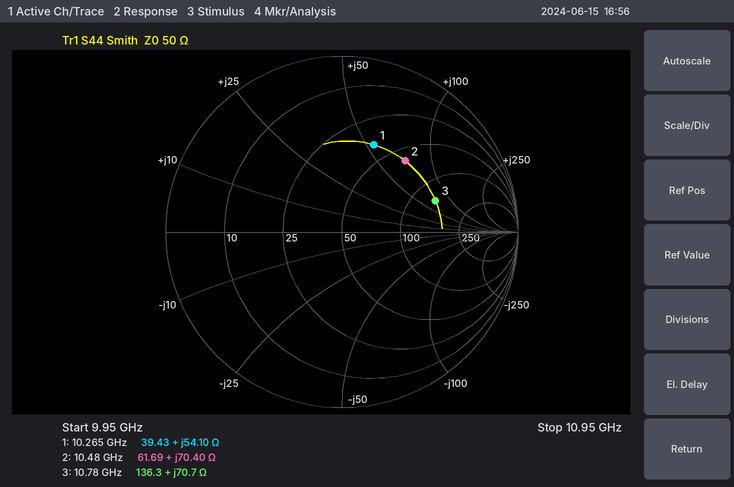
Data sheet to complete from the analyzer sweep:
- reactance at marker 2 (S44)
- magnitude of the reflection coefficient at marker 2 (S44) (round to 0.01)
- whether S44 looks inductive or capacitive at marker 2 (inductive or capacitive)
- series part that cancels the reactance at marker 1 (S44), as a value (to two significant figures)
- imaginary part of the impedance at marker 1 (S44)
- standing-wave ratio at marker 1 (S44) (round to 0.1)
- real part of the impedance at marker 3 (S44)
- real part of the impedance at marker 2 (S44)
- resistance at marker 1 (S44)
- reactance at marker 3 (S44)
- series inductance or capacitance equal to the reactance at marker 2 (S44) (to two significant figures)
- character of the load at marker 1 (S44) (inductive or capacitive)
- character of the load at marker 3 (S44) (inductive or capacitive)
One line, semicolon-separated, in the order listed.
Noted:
+70.40 Ω; 0.54; inductive; 290 fF; +54.10 Ω; 3.2; 136.3 Ω; 61.69 Ω; 39.43 Ω; +70.7 Ω; 1.1 nH; inductive; inductive
